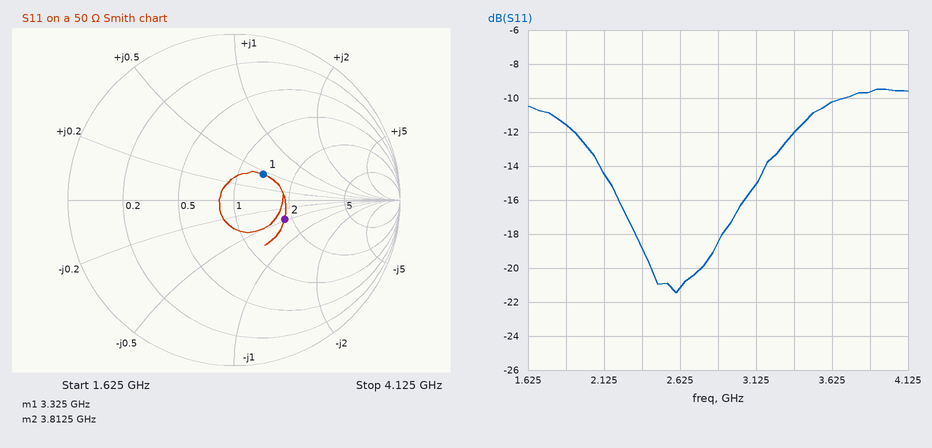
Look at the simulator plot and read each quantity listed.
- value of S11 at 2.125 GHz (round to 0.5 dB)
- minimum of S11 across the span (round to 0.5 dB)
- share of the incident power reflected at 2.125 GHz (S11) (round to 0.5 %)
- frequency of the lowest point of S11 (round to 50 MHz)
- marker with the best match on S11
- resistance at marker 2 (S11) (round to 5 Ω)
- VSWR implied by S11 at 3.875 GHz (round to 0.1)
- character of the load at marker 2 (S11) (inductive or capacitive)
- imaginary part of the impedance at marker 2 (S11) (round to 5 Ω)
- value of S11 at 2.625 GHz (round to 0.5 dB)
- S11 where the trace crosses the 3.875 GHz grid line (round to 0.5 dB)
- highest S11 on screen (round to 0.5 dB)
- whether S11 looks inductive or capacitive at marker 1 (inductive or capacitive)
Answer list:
-14.5 dB
-21.5 dB
3.5 %
2.60 GHz
marker 1
90 Ω
2.0
capacitive
-25 Ω
-21.0 dB
-9.5 dB
-9.5 dB
inductive
